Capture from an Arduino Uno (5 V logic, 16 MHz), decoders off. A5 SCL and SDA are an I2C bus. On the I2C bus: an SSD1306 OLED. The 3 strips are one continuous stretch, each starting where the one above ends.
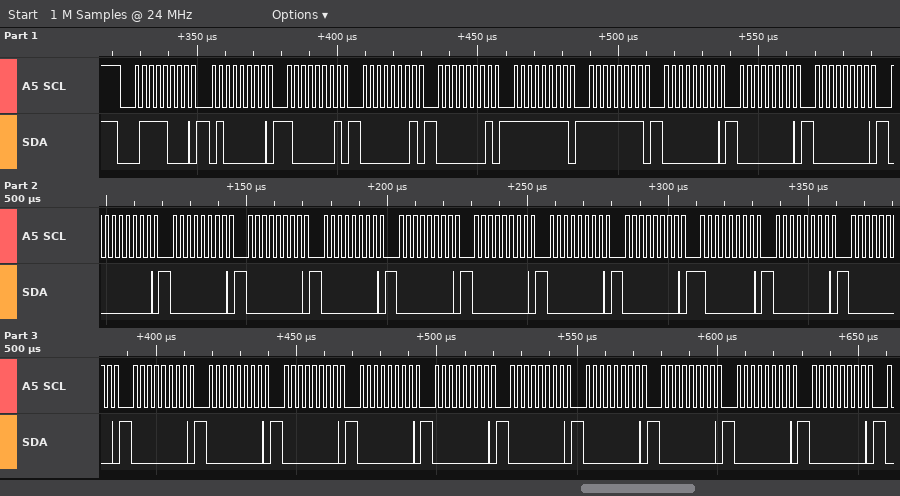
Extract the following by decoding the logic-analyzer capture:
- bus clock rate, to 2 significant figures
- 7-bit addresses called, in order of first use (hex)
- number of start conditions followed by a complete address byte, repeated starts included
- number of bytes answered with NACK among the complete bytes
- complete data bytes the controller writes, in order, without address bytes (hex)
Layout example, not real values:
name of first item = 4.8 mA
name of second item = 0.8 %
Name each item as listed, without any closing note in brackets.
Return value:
bus clock rate, to 2 significant figures = 400 kHz
7-bit addresses called, in order of first use = 0x3C
number of start conditions followed by a complete address byte, repeated starts included = 1
number of bytes answered with NACK among the complete bytes = 0
complete data bytes the controller writes, in order, without address bytes = 40 81 01 01 FF FF 00 00 00 00 00 00 00 00 00 00 00 80 00 00 00 00 00 00 00 00 00 00 00 00
